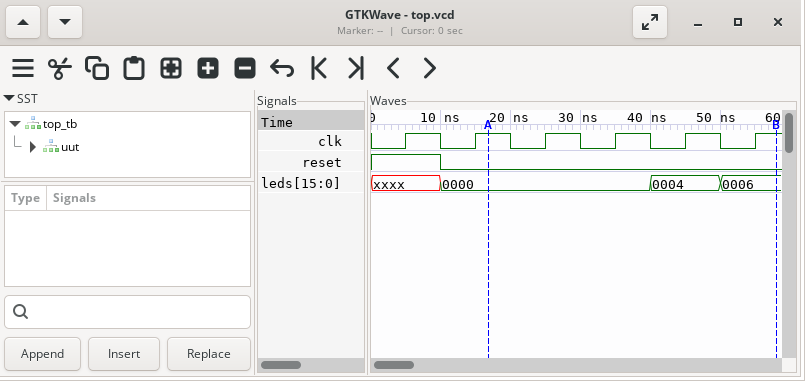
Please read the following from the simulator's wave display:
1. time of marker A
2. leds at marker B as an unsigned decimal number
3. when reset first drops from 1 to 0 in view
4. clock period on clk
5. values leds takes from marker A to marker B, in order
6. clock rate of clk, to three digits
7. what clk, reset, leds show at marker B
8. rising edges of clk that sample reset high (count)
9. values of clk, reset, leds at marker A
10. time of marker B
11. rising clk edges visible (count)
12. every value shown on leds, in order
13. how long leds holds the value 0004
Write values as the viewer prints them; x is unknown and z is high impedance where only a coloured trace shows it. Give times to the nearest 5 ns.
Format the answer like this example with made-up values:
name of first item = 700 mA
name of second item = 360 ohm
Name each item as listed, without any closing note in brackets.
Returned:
time of marker A = 15 ns
leds at marker B as an unsigned decimal number = 6
when reset first drops from 1 to 0 in view = 10 ns
clock period on clk = 10 ns
values leds takes from marker A to marker B, in order = 0000, 0004, 0006
clock rate of clk, to three digits = 100 MHz
what clk, reset, leds show at marker B = clk=1, reset=0, leds=0006
rising edges of clk that sample reset high = 1
values of clk, reset, leds at marker A = clk=1, reset=0, leds=0000
time of marker B = 60 ns
rising clk edges visible = 6
every value shown on leds, in order = xxxx, 0000, 0004, 0006
how long leds holds the value 0004 = 10 ns
